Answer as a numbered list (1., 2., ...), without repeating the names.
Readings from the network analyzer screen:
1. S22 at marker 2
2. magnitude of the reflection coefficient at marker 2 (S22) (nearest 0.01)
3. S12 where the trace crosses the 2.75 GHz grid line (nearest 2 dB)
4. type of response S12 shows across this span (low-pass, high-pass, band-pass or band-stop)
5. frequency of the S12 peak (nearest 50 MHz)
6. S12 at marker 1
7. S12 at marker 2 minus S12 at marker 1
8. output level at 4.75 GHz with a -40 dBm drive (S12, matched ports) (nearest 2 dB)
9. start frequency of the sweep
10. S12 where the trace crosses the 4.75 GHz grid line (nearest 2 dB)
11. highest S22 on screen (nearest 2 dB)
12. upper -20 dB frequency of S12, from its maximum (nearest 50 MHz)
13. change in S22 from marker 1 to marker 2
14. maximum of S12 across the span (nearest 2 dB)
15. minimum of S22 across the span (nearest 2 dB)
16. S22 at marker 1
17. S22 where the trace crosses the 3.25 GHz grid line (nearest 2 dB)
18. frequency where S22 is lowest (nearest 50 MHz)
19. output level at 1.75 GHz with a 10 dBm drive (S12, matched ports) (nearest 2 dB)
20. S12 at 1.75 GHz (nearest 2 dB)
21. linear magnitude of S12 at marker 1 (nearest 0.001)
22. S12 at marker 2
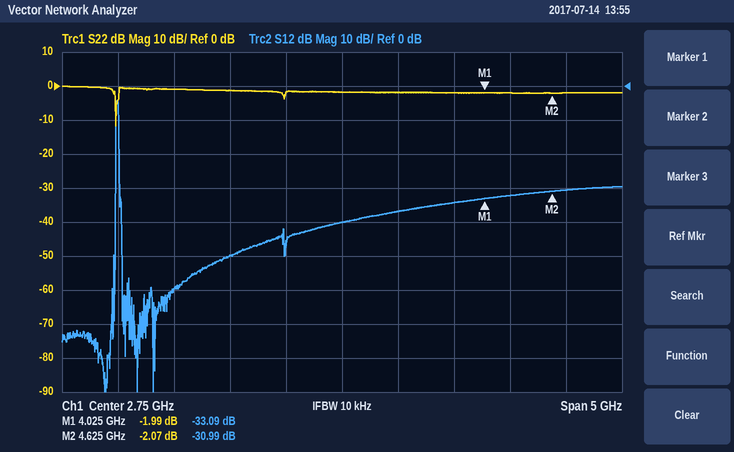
1. -2.07 dB
2. 0.79
3. -40 dB
4. band-pass
5. 750 MHz
6. -33.09 dB
7. 2.10 dB
8. -70 dBm
9. 250 MHz
10. -30 dB
11. 0 dB
12. 750 MHz
13. -0.08 dB
14. -4 dB
15. -12 dB
16. -1.99 dB
17. -2 dB
18. 750 MHz
19. -40 dBm
20. -50 dB
21. 0.022
22. -30.99 dB
